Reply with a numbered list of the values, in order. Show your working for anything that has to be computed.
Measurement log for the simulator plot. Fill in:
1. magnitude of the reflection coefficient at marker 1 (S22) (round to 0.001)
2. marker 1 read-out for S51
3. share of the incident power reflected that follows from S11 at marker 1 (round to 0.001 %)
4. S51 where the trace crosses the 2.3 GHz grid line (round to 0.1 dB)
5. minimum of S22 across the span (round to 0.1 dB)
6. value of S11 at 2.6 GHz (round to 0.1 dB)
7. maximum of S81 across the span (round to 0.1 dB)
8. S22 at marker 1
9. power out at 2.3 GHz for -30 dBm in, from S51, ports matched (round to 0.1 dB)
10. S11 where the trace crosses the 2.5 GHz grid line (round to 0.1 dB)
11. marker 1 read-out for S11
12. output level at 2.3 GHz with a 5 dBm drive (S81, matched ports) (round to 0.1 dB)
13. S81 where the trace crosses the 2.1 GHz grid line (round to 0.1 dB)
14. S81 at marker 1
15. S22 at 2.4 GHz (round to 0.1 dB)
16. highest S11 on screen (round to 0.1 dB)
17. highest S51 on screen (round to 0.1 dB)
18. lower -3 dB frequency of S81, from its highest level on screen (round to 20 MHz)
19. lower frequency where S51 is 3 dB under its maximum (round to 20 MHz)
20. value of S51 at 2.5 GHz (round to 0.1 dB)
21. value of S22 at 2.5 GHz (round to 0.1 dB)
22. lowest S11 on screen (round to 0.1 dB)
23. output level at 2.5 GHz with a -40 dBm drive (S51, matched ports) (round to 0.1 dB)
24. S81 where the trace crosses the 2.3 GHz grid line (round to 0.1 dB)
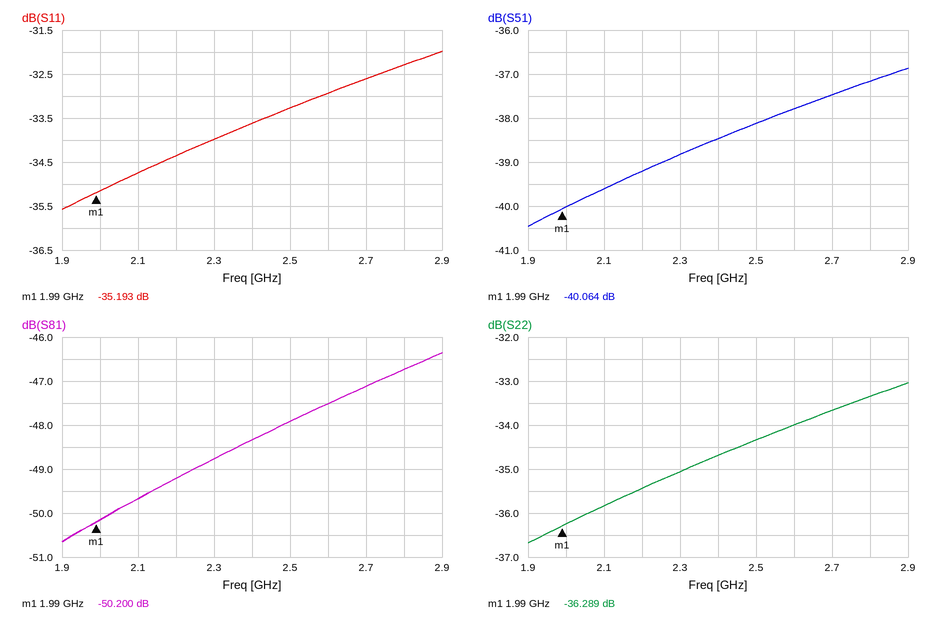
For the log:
1. 10^(-36.289/20) ≈ 0.015
2. -40.064 dB
3. 10^(-35.193/10) ≈ 0.030 %
4. -38.8 dB
5. -36.7 dB
6. -32.9 dB
7. -46.4 dB
8. -36.289 dB
9. -30 dBm + (-38.8 dB) = -68.8 dBm
10. -33.3 dB
11. -35.193 dB
12. 5 dBm + (-48.8 dB) = -43.8 dBm
13. -49.7 dB
14. -50.200 dB
15. -34.7 dB
16. -32.0 dB
17. -36.9 dB
18. 2.16 GHz
19. 2.04 GHz
20. -38.1 dB
21. -34.3 dB
22. -35.6 dB
23. -40 dBm + (-38.1 dB) = -78.1 dBm
24. -48.8 dB
